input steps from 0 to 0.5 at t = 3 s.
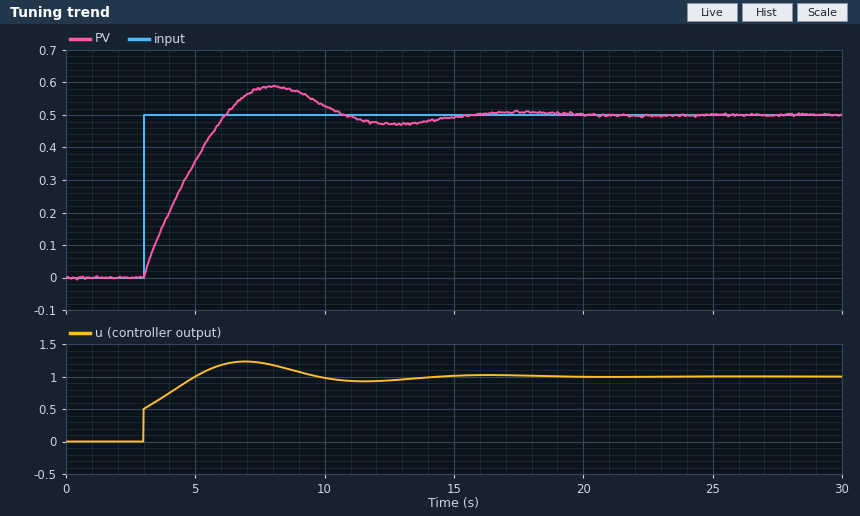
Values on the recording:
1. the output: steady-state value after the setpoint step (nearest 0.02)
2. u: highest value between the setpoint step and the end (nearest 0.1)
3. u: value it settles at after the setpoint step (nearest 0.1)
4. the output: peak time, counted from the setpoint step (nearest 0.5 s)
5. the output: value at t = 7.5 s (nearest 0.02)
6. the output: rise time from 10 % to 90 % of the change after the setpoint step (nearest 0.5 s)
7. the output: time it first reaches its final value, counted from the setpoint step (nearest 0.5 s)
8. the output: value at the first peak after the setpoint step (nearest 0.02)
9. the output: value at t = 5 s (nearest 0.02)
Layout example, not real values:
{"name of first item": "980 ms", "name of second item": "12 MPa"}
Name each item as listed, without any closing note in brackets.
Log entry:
{"the output: steady-state value after the setpoint step": "0.50", "u: highest value between the setpoint step and the end": "1.2", "u: value it settles at after the setpoint step": "1.0", "the output: peak time, counted from the setpoint step": "5.0 s", "the output: value at t = 7.5 s": "0.58", "the output: rise time from 10 % to 90 % of the change after the setpoint step": "2.5 s", "the output: time it first reaches its final value, counted from the setpoint step": "3.0 s", "the output: value at the first peak after the setpoint step": "0.58", "the output: value at t = 5 s": "0.36"}
